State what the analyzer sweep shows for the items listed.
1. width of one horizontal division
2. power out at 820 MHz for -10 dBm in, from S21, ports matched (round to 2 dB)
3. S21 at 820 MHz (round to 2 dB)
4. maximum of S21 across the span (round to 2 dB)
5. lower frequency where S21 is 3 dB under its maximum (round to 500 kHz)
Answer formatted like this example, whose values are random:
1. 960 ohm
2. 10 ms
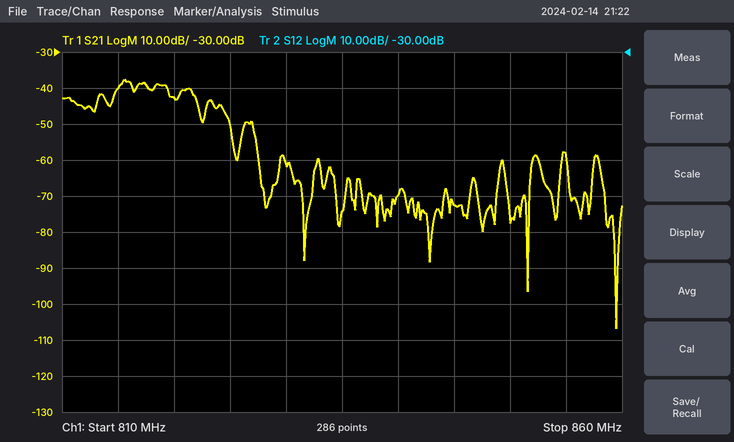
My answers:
1. 5 MHz
2. -52 dBm
3. -42 dB
4. -38 dB
5. 815.0 MHz
